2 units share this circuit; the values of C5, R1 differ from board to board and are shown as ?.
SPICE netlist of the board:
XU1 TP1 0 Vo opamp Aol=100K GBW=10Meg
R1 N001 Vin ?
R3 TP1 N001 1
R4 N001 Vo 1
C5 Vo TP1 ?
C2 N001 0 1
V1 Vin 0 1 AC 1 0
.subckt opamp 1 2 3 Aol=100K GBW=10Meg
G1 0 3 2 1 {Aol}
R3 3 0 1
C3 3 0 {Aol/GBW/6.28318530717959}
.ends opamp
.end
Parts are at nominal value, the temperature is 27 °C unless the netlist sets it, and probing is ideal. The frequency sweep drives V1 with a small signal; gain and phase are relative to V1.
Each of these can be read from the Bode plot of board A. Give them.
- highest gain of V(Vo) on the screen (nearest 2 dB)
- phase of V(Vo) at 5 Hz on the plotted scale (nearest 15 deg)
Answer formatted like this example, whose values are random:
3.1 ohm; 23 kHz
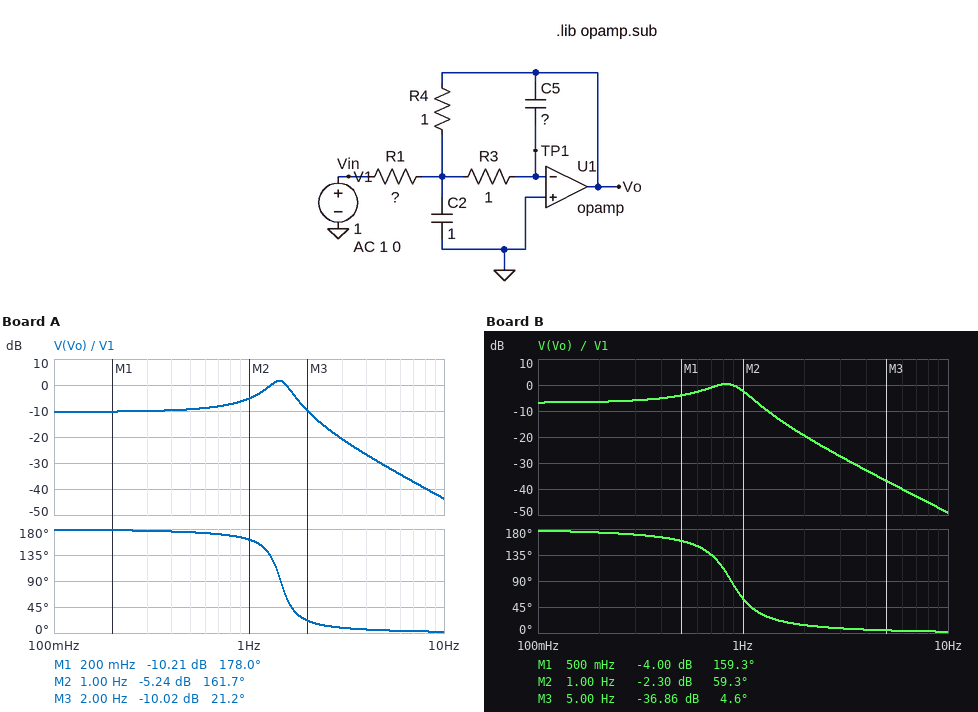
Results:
2 dB; 0 deg
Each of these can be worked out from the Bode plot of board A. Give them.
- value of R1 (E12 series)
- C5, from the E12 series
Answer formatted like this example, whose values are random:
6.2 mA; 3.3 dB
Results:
3.3 Ω; 12 mF
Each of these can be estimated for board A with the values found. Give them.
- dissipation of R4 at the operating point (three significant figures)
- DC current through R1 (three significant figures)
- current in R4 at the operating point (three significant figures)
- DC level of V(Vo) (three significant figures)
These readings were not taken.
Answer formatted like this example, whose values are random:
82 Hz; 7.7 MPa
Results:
91.8 mW; 303 mA; 303 mA; -303 mV
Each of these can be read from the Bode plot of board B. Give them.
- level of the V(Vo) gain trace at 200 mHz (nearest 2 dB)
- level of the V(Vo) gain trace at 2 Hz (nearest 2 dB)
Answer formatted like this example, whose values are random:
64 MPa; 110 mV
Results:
-6 dB; -20 dB
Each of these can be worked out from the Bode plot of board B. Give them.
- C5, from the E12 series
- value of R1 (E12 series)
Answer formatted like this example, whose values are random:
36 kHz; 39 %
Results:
33 mF; 2.2 Ω
